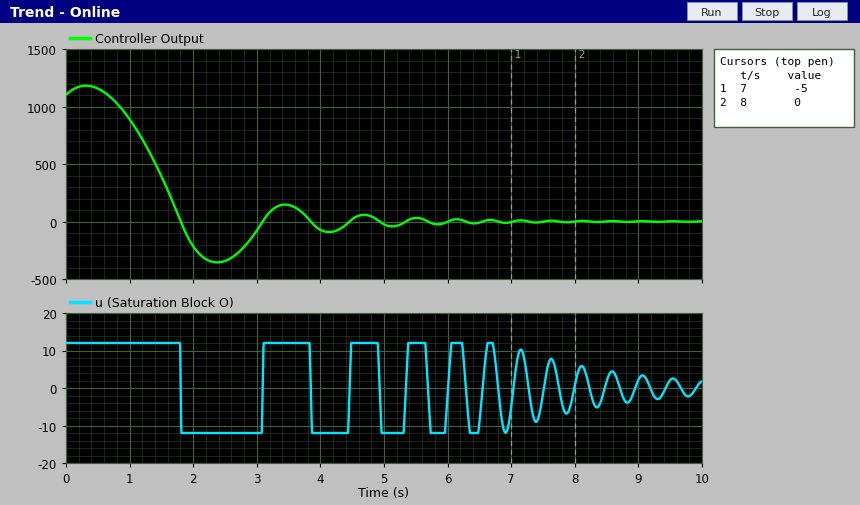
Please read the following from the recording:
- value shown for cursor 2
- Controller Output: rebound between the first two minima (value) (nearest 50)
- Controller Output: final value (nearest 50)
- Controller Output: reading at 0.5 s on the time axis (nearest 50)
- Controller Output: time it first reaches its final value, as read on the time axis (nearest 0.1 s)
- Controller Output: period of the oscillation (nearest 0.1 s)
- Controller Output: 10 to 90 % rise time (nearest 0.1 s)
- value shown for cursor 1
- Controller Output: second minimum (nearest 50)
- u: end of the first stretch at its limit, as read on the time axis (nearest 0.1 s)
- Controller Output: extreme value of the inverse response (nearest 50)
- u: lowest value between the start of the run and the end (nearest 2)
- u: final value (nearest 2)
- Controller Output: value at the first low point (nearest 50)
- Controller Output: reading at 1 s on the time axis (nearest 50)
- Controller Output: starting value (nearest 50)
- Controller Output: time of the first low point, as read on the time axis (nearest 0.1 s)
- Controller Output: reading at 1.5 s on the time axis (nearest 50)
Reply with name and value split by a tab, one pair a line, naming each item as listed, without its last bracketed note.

value shown for cursor 2	0
Controller Output: rebound between the first two minima (value)	150
Controller Output: final value	0
Controller Output: reading at 0.5 s on the time axis	1150
Controller Output: time it first reaches its final value, as read on the time axis	1.8 s
Controller Output: period of the oscillation	1.8 s
Controller Output: 10 to 90 % rise time	0.9 s
value shown for cursor 1	-5
Controller Output: second minimum	-100
u: end of the first stretch at its limit, as read on the time axis	1.8 s
Controller Output: extreme value of the inverse response	1200
u: lowest value between the start of the run and the end	-12
u: final value	0
Controller Output: value at the first low point	-350
Controller Output: reading at 1 s on the time axis	900
Controller Output: starting value	1100
Controller Output: time of the first low point, as read on the time axis	2.4 s
Controller Output: reading at 1.5 s on the time axis	400
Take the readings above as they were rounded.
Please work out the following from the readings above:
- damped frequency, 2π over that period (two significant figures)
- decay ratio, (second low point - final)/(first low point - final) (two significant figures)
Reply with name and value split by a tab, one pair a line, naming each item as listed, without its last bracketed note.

damped frequency, 2π over that period	3.5 rad/s
decay ratio, (second low point - final)/(first low point - final)	0.29
